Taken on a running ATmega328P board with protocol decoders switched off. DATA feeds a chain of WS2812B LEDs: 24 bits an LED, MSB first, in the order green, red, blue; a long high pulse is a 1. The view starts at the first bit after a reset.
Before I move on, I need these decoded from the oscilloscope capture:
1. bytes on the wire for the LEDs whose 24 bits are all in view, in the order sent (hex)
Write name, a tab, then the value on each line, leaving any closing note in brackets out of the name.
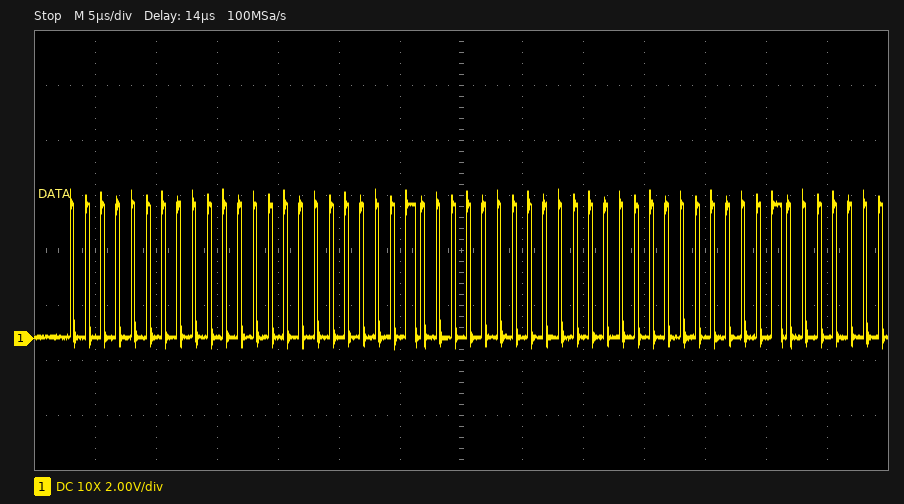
bytes on the wire for the LEDs whose 24 bits are all in view, in the order sent	00 00 02 00 00 02
